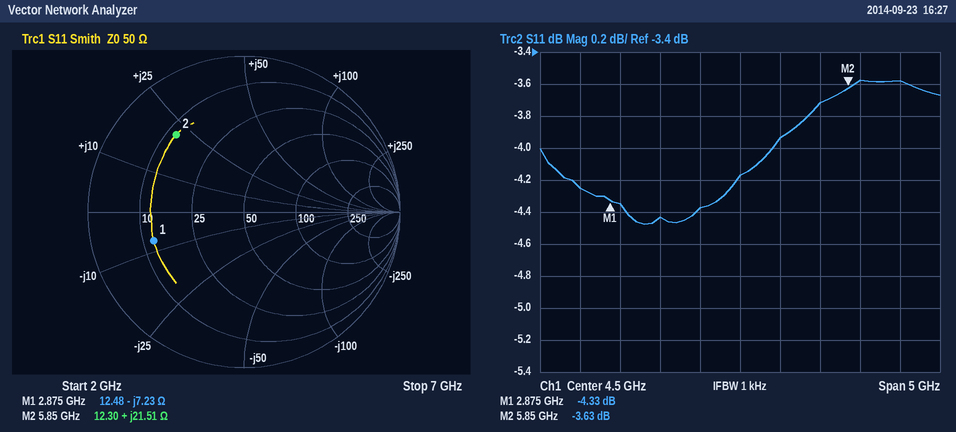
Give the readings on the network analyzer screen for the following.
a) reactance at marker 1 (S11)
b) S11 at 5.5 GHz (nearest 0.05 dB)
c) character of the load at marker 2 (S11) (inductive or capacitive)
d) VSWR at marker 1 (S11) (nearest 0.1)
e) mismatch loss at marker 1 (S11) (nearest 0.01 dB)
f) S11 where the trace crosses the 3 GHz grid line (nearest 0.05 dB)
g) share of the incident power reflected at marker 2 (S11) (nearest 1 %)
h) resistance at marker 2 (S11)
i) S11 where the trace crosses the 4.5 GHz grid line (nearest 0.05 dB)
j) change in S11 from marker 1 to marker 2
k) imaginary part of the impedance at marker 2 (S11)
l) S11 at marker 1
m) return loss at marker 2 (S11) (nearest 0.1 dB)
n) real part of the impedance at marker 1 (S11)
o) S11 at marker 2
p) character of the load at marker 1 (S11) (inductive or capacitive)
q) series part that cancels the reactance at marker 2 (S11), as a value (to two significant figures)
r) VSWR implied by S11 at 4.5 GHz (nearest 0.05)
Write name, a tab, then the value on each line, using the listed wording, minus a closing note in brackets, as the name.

reactance at marker 1	-7.23 Ω
S11 at 5.5 GHz	-3.70 dB
character of the load at marker 2 (S11)	inductive
VSWR at marker 1 (S11)	4.1
mismatch loss at marker 1 (S11)	2.00 dB
S11 where the trace crosses the 3 GHz grid line	-4.35 dB
share of the incident power reflected at marker 2 (S11)	43 %
resistance at marker 2	12.30 Ω
S11 where the trace crosses the 4.5 GHz grid line	-4.15 dB
change in S11 from marker 1 to marker 2	0.70 dB
imaginary part of the impedance at marker 2	+21.51 Ω
S11 at marker 1	-4.33 dB
return loss at marker 2 (S11)	3.6 dB
real part of the impedance at marker 1	12.48 Ω
S11 at marker 2	-3.63 dB
character of the load at marker 1 (S11)	capacitive
series part that cancels the reactance at marker 2 (S11), as a value	1.3 pF
VSWR implied by S11 at 4.5 GHz	4.25
